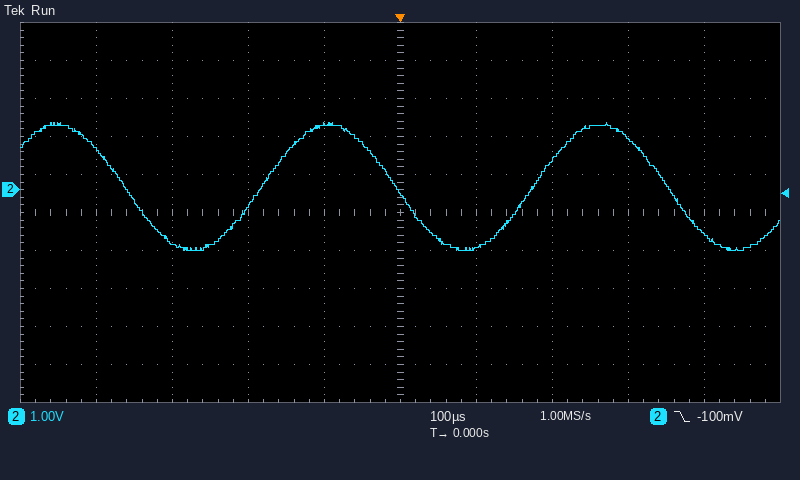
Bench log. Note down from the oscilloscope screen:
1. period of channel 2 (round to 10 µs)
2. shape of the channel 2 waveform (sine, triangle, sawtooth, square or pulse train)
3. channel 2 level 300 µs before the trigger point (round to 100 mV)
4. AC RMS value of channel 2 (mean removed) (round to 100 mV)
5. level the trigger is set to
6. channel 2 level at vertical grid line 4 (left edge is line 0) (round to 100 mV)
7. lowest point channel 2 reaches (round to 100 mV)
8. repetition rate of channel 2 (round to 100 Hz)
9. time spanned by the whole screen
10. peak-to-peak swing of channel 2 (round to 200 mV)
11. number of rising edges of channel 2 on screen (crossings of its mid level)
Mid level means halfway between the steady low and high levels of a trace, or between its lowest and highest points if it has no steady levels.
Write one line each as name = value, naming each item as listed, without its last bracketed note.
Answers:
period of channel 2 = 360 µs
shape of the channel 2 waveform = sine
channel 2 level 300 µs before the trigger point = -1.4 V
AC RMS value of channel 2 (mean removed) = 1.2 V
level the trigger is set to = -100 mV
channel 2 level at vertical grid line 4 (left edge is line 0) = 1.7 V
lowest point channel 2 reaches = -1.6 V
repetition rate of channel 2 = 2.8 kHz
time spanned by the whole screen = 1 ms
peak-to-peak swing of channel 2 = 3.4 V
number of rising edges of channel 2 on screen = 2
